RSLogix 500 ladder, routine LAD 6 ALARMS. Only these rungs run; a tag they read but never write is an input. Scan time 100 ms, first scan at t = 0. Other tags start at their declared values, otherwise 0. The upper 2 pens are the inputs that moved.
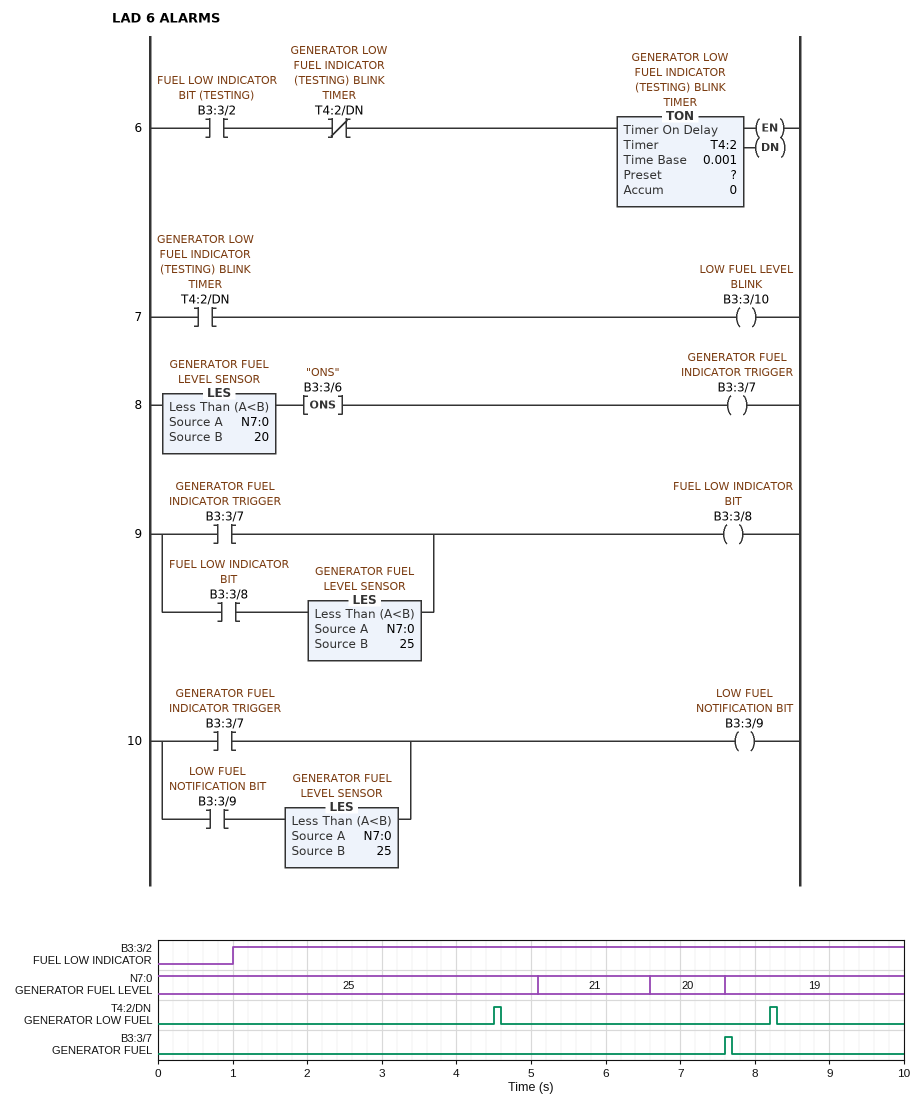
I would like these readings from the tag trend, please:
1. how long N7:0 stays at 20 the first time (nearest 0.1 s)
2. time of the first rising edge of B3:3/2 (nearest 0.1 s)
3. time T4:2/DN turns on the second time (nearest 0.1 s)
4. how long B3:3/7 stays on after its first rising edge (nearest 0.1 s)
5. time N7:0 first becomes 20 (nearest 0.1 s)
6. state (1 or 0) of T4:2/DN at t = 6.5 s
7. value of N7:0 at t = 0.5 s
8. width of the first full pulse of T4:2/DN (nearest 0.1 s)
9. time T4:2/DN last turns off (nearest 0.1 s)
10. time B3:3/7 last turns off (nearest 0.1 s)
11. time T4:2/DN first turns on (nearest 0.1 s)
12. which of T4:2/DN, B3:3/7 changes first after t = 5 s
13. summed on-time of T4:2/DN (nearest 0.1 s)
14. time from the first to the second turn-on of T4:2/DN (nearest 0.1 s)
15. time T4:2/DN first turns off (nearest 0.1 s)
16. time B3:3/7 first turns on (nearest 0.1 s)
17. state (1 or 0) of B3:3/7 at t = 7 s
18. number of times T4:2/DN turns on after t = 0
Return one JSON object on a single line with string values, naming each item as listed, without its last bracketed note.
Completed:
{"how long N7:0 stays at 20 the first time": "1.0 s", "time of the first rising edge of B3:3/2": "1.0 s", "time T4:2/DN turns on the second time": "8.2 s", "how long B3:3/7 stays on after its first rising edge": "0.1 s", "time N7:0 first becomes 20": "6.6 s", "state (1 or 0) of T4:2/DN at t = 6.5 s": "0", "value of N7:0 at t = 0.5 s": "25", "width of the first full pulse of T4:2/DN": "0.1 s", "time T4:2/DN last turns off": "8.3 s", "time B3:3/7 last turns off": "7.7 s", "time T4:2/DN first turns on": "4.5 s", "which of T4:2/DN, B3:3/7 changes first after t = 5 s": "B3:3/7", "summed on-time of T4:2/DN": "0.2 s", "time from the first to the second turn-on of T4:2/DN": "3.7 s", "time T4:2/DN first turns off": "4.6 s", "time B3:3/7 first turns on": "7.6 s", "state (1 or 0) of B3:3/7 at t = 7 s": "0", "number of times T4:2/DN turns on after t = 0": "2"}
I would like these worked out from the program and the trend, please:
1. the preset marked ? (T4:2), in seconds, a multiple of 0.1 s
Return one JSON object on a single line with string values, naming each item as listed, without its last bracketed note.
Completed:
{"the preset marked ? (T4:2), in seconds, a multiple of 0.1 s": "3.5 s"}
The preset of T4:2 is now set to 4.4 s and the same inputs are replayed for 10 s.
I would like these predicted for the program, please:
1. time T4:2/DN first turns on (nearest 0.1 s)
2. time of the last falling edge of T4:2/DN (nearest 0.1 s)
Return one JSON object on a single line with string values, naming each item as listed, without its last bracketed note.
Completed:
{"time T4:2/DN first turns on": "5.4 s", "time of the last falling edge of T4:2/DN": "5.5 s"}
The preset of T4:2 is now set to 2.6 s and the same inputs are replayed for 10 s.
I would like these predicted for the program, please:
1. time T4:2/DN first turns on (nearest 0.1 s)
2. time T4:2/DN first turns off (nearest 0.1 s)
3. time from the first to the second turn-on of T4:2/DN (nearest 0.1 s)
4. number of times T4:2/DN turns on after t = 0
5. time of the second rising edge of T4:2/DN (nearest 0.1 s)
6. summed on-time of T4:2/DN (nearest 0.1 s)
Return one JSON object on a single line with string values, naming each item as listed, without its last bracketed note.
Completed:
{"time T4:2/DN first turns on": "3.6 s", "time T4:2/DN first turns off": "3.7 s", "time from the first to the second turn-on of T4:2/DN": "2.8 s", "number of times T4:2/DN turns on after t = 0": "3", "time of the second rising edge of T4:2/DN": "6.4 s", "summed on-time of T4:2/DN": "0.3 s"}
